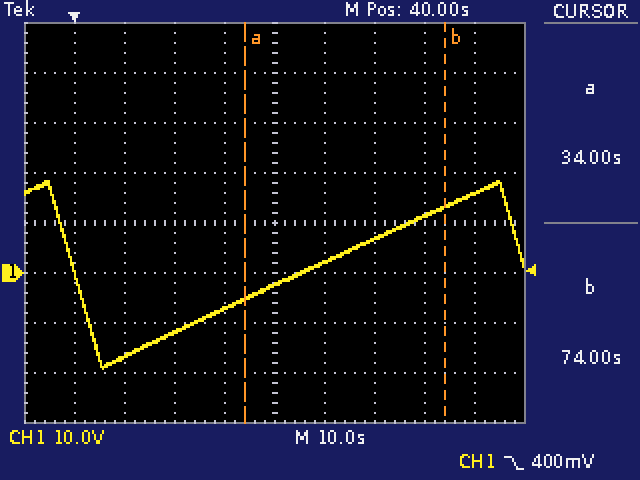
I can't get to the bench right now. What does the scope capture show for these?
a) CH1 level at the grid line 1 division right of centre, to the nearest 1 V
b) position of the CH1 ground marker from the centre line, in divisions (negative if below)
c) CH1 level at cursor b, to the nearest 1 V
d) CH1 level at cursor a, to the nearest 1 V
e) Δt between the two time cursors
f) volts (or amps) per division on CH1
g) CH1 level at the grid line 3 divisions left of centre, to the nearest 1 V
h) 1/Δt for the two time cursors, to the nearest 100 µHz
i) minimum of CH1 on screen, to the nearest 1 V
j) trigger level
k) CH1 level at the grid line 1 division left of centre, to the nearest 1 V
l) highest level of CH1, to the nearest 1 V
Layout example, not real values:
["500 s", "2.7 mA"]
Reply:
["2 V", "-1.0 div", "13 V", "-5 V", "40 s", "10 V", "-17 V", "25.0 mHz", "-19 V", "400 mV", "-7 V", "18 V"]
